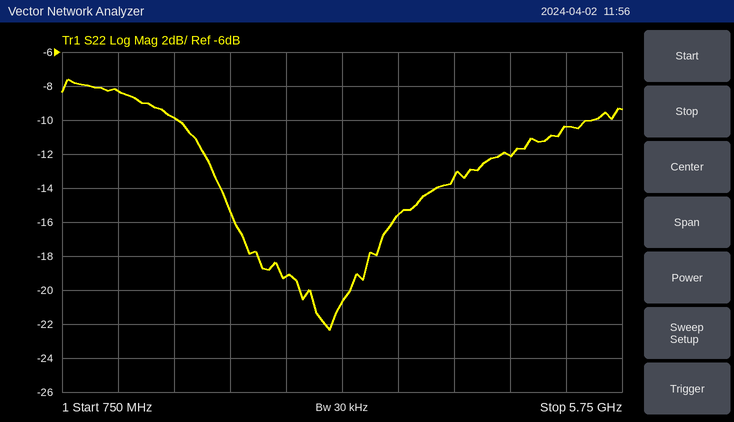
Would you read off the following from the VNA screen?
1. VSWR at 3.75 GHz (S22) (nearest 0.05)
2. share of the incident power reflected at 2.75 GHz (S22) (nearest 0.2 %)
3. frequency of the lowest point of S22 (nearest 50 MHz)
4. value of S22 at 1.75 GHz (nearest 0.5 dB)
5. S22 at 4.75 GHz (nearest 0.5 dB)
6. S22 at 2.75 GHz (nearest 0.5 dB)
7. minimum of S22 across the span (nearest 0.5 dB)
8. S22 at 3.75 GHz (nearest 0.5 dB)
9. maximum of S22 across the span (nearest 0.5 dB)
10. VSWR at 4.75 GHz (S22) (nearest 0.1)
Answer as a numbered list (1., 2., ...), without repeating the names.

1. 1.40
2. 1.2 %
3. 3.15 GHz
4. -10.0 dB
5. -12.0 dB
6. -19.0 dB
7. -22.5 dB
8. -15.5 dB
9. -7.5 dB
10. 1.7
